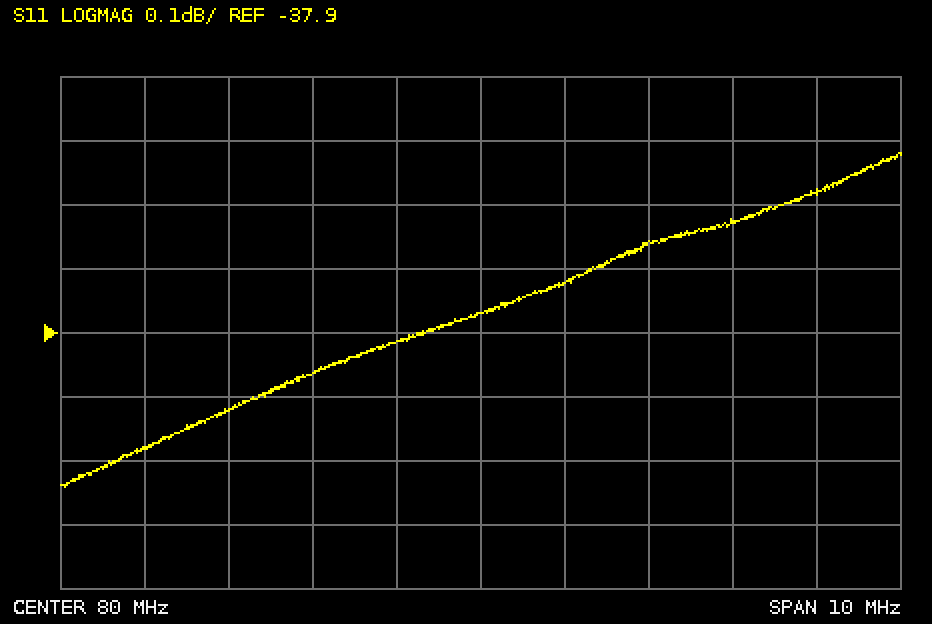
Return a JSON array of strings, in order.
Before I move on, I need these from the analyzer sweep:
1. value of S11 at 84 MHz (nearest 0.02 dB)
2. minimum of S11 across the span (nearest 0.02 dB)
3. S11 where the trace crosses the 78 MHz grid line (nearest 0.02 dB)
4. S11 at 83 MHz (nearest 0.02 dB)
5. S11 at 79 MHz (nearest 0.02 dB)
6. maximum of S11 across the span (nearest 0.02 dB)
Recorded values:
["-37.68 dB", "-38.14 dB", "-37.96 dB", "-37.72 dB", "-37.92 dB", "-37.62 dB"]
